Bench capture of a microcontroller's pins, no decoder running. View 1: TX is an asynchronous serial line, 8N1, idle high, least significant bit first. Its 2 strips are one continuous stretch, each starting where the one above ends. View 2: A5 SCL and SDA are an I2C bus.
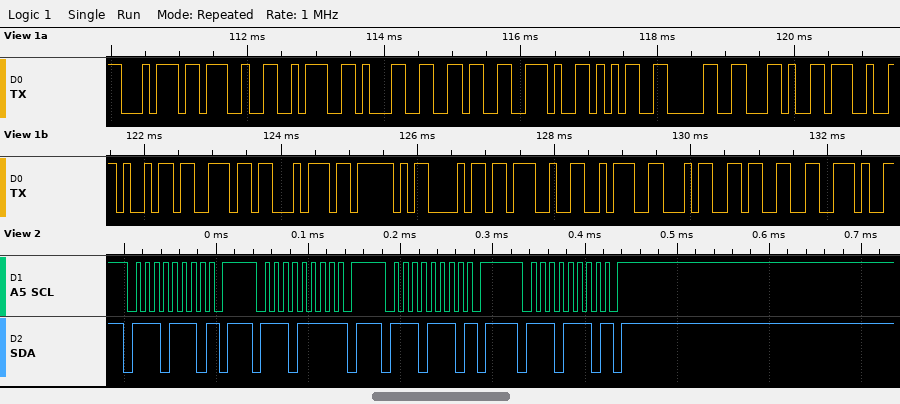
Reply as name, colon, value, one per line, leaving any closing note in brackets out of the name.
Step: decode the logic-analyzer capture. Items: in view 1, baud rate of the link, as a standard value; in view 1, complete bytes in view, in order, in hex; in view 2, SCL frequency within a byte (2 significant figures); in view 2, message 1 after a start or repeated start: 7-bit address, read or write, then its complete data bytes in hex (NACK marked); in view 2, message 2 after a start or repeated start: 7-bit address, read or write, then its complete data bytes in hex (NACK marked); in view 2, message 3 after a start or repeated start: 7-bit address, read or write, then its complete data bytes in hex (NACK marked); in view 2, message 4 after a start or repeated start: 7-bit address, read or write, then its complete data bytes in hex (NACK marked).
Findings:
in view 1, baud rate of the link, as a standard value: 9600 baud
in view 1, complete bytes in view, in order, in hex: 74 27 3A 31 36 2E 35 30 2C 27 69 6E 74 5F 68 27 3A 34 33 2E
in view 2, SCL frequency within a byte: 100 kHz
in view 2, message 1 after a start or repeated start: 7-bit address, read or write, then its complete data bytes in hex: 0x77 write NACK
in view 2, message 2 after a start or repeated start: 7-bit address, read or write, then its complete data bytes in hex: 0x77 read NACK
in view 2, message 3 after a start or repeated start: 7-bit address, read or write, then its complete data bytes in hex: 0x77 write NACK
in view 2, message 4 after a start or repeated start: 7-bit address, read or write, then its complete data bytes in hex: 0x77 write NACK
